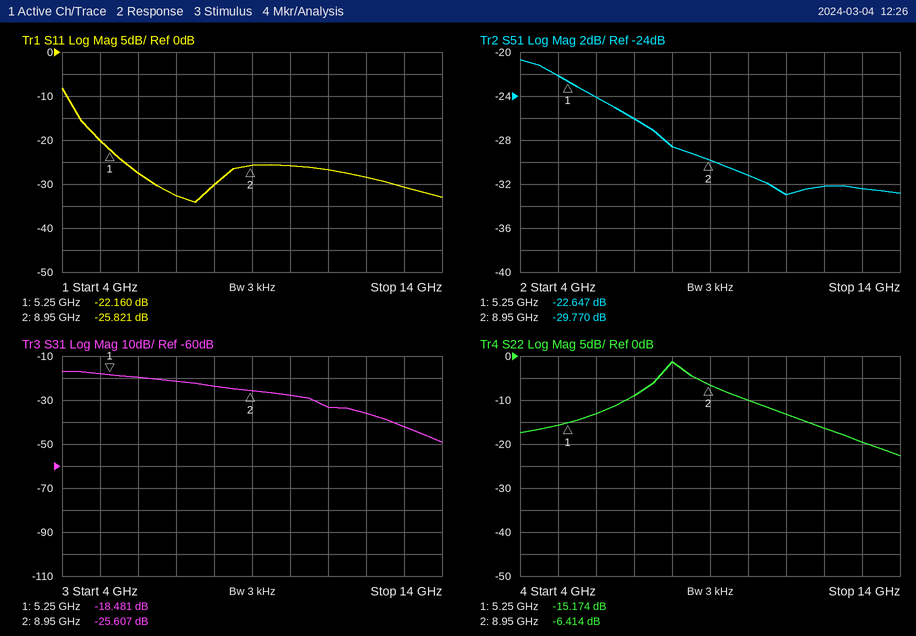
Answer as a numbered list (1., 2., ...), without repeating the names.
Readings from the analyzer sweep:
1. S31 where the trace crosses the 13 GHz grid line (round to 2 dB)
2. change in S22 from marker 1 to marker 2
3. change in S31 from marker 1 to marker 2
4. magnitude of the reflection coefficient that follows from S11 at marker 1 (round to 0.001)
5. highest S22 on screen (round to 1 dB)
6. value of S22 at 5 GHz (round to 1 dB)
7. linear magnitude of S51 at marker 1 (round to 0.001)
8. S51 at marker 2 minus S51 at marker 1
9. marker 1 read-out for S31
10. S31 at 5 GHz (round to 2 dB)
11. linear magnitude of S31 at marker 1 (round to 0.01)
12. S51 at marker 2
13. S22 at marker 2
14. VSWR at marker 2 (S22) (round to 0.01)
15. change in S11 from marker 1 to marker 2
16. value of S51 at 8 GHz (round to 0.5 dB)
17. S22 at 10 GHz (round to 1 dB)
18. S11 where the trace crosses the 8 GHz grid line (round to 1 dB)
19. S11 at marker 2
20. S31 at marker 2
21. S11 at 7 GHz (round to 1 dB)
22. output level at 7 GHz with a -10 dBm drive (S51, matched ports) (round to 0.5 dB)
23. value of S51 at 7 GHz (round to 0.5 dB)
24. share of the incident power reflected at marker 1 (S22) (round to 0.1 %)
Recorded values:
1. -42 dB
2. 8.760 dB
3. -7.126 dB
4. 0.078
5. -1 dB
6. -16 dB
7. 0.074
8. -7.123 dB
9. -18.481 dB
10. -18 dB
11. 0.12
12. -29.770 dB
13. -6.414 dB
14. 2.83
15. -3.661 dB
16. -28.5 dB
17. -10 dB
18. -30 dB
19. -25.821 dB
20. -25.607 dB
21. -33 dB
22. -36.0 dBm
23. -26.0 dB
24. 3.0 %
